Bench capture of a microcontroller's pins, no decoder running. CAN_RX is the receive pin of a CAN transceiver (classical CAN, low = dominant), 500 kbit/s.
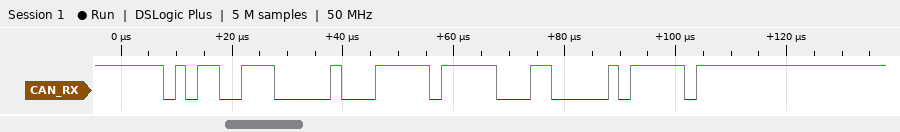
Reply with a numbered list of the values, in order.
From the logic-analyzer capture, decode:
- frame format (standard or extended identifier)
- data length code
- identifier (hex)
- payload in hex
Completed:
1. standard
2. 1
3. 0x59C
4. FF
